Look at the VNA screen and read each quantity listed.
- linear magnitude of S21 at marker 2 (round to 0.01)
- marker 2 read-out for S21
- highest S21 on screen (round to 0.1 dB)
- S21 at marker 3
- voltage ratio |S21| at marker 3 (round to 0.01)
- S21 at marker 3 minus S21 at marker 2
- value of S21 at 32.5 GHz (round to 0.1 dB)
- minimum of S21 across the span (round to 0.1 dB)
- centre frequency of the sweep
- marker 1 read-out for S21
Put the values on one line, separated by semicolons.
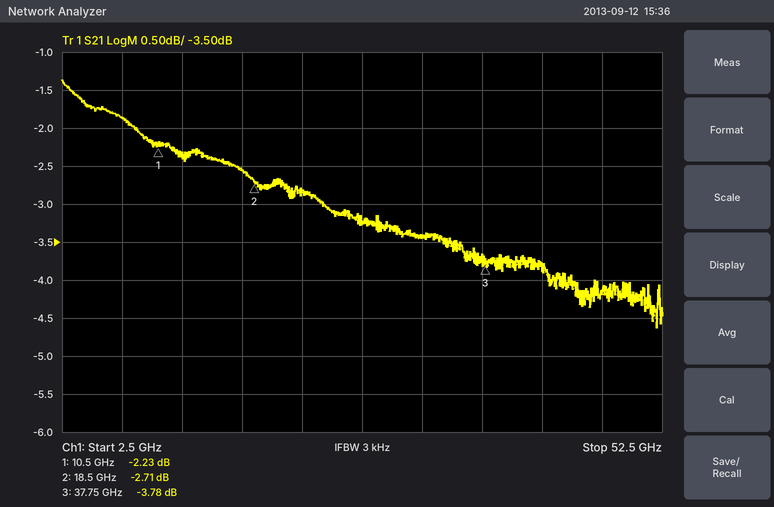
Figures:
0.73; -2.71 dB; -1.4 dB; -3.78 dB; 0.65; -1.07 dB; -3.4 dB; -4.6 dB; 27.5 GHz; -2.23 dB
